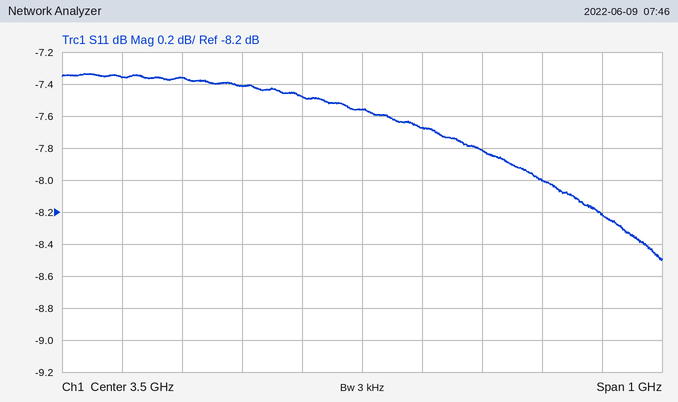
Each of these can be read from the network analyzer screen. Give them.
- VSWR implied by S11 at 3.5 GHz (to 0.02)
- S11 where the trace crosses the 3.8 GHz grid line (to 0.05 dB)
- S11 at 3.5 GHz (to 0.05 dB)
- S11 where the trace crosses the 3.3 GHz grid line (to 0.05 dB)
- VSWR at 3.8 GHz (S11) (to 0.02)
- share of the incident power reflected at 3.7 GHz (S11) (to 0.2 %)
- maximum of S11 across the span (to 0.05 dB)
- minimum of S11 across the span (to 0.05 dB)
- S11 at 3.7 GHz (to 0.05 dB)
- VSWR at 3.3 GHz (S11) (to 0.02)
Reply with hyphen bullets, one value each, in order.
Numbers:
- 2.44
- -8.00 dB
- -7.55 dB
- -7.40 dB
- 2.32
- 16.6 %
- -7.35 dB
- -8.50 dB
- -7.80 dB
- 2.48
